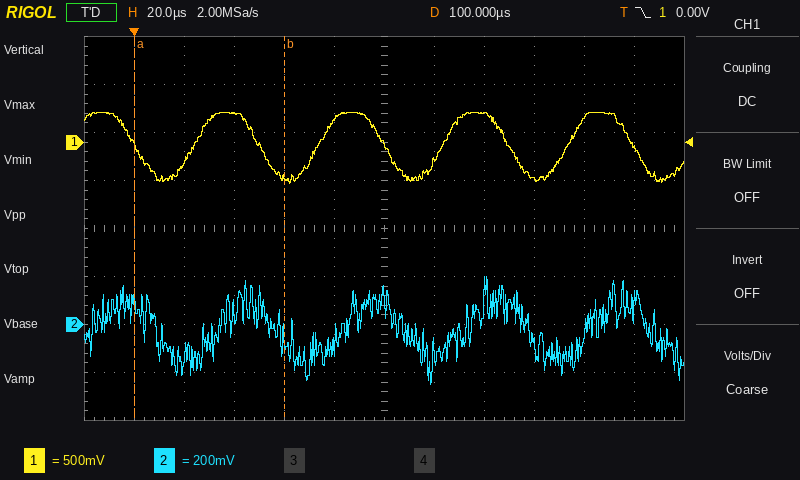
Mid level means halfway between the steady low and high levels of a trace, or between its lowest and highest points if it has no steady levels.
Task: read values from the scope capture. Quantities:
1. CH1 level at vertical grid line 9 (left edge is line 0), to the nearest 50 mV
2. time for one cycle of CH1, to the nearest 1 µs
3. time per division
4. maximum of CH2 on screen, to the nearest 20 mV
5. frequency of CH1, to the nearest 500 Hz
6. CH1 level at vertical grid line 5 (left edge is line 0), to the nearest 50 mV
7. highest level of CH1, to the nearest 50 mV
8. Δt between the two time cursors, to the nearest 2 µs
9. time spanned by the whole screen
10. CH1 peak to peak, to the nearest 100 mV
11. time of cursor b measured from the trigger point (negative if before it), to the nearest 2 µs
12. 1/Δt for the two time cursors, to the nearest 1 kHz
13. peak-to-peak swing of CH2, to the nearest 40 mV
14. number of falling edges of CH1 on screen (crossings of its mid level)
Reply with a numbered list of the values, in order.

1. -400 mV
2. 50 µs
3. 20 µs
4. 200 mV
5. 20.0 kHz
6. 250 mV
7. 300 mV
8. 60 µs
9. 240 µs
10. 700 mV
11. +60 µs
12. 17 kHz
13. 440 mV
14. 5
